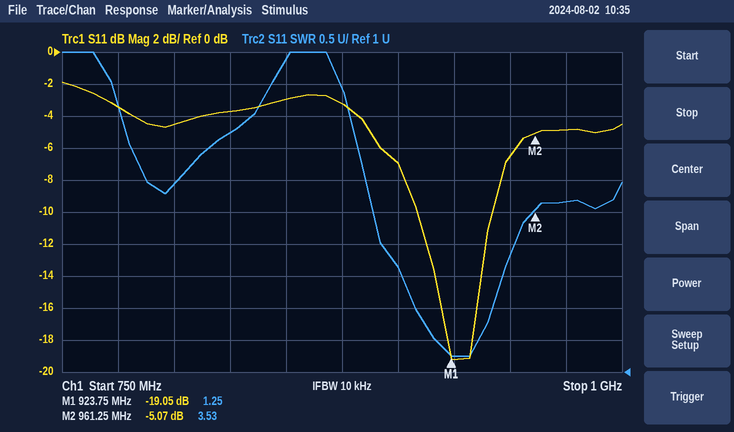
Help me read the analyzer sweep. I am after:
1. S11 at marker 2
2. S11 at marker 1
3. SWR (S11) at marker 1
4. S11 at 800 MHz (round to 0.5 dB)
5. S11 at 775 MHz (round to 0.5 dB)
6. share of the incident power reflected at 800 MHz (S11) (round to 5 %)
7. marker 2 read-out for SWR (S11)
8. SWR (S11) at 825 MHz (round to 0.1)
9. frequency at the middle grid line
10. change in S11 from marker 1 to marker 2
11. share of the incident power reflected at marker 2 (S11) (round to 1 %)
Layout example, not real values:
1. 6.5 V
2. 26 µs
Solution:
1. -5.07 dB
2. -19.05 dB
3. 1.25
4. -4.5 dB
5. -3.5 dB
6. 35 %
7. 3.53
8. 4.7
9. 875 MHz
10. 13.98 dB
11. 31 %
